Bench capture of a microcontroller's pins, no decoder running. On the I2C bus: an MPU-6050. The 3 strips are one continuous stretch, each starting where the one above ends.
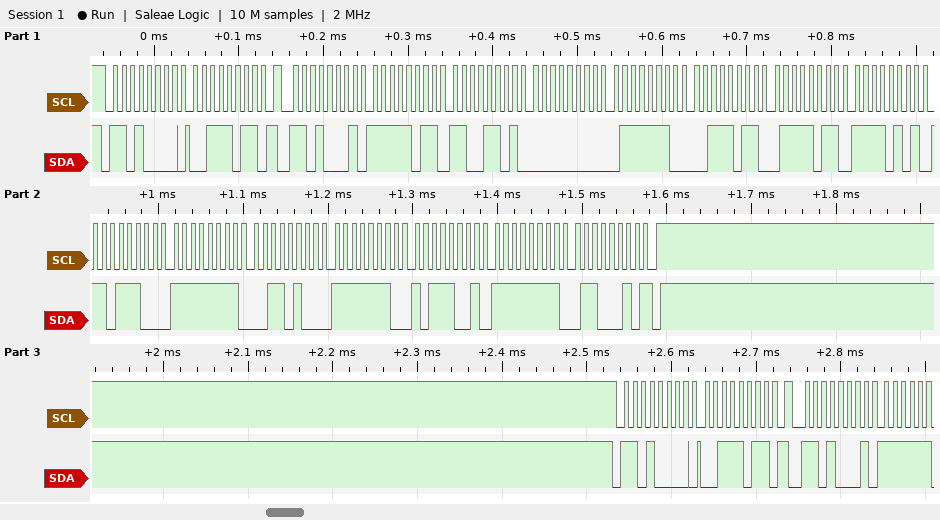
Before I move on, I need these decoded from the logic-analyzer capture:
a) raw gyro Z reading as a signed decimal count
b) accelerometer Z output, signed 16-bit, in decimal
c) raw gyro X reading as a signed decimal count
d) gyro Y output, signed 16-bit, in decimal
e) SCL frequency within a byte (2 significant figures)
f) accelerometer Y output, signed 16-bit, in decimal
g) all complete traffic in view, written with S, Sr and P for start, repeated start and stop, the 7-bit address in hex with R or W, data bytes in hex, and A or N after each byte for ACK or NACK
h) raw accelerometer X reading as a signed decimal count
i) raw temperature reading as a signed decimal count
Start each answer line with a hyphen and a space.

- -158
- 15227
- -204
- -327
- 100 kHz
- 126
- S 68W A 3B A Sr 68R A FB A CD A 00 A 7E A 3B A 7B A F5 A DC A FF A 34 A FE A B9 A FF A 62 N P S 68W A 3B A Sr 68R A
- -1075
- -2596
